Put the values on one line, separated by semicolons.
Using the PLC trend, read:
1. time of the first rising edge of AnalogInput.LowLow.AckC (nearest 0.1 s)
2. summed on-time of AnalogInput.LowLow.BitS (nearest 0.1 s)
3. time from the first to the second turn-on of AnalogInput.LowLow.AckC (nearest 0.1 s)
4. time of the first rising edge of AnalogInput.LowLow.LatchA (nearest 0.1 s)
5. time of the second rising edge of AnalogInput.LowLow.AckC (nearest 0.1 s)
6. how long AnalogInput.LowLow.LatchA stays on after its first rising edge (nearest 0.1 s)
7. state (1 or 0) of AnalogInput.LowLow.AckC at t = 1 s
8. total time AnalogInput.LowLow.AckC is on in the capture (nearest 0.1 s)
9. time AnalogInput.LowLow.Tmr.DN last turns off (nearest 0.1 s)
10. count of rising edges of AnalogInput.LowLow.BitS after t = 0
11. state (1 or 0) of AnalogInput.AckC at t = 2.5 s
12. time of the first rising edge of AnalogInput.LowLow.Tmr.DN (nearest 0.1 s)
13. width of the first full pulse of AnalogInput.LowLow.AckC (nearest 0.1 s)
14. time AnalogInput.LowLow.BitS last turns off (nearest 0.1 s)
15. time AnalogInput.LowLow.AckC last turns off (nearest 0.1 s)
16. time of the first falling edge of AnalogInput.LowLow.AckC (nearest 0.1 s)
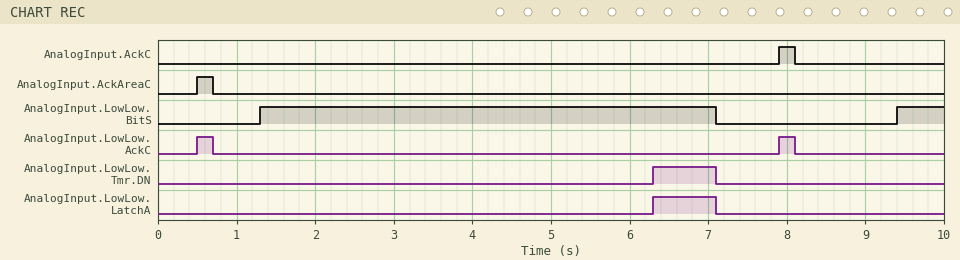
0.5 s; 6.4 s; 7.4 s; 6.3 s; 7.9 s; 0.8 s; 0; 0.4 s; 7.1 s; 2; 0; 6.3 s; 0.2 s; 7.1 s; 8.1 s; 0.7 s
